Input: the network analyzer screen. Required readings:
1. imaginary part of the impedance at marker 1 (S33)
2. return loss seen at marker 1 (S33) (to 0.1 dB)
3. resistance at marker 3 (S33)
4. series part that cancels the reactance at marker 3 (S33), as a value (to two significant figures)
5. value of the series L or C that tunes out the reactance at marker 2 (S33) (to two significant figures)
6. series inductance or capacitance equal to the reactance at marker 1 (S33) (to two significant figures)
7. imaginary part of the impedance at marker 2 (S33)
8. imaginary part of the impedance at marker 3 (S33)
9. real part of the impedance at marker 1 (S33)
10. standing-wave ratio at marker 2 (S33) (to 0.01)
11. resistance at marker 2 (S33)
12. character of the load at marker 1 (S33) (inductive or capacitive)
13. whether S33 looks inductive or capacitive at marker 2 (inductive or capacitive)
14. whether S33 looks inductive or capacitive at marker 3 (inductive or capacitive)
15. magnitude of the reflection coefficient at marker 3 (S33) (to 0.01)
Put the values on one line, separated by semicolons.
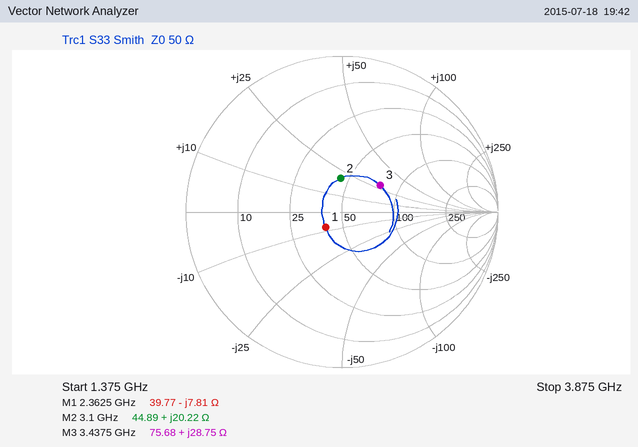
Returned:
-7.81 Ω; 16.9 dB; 75.68 Ω; 1.6 pF; 2.5 pF; 8.6 pF; +20.22 Ω; +28.75 Ω; 39.77 Ω; 1.55; 44.89 Ω; capacitive; inductive; inductive; 0.30
